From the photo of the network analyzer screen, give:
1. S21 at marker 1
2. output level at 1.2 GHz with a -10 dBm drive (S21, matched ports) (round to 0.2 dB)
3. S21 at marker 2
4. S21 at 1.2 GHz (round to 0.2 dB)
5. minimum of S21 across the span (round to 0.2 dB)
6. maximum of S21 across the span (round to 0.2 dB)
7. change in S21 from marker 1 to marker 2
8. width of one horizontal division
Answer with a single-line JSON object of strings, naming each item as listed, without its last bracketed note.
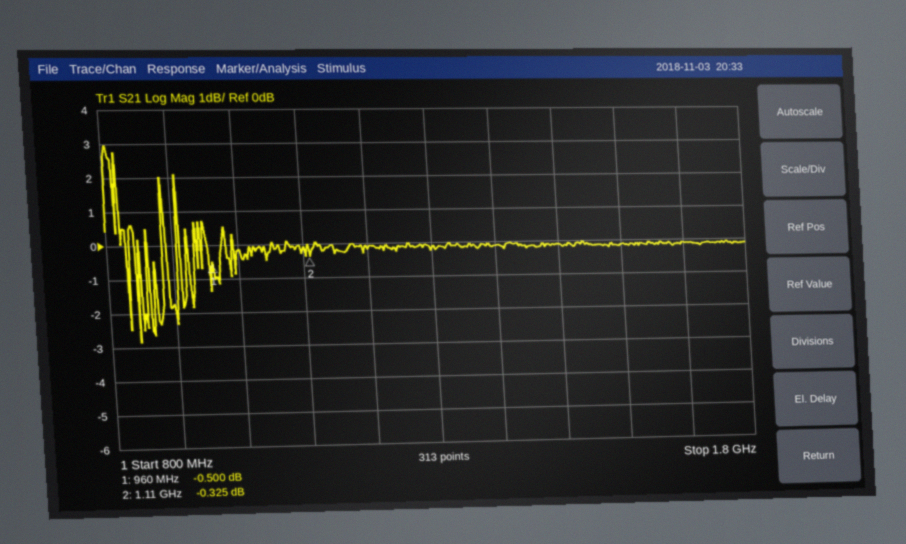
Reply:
{"S21 at marker 1": "-0.500 dB", "output level at 1.2 GHz with a -10 dBm drive (S21, matched ports)": "-10.2 dBm", "S21 at marker 2": "-0.325 dB", "S21 at 1.2 GHz": "-0.2 dB", "minimum of S21 across the span": "-2.8 dB", "maximum of S21 across the span": "3.0 dB", "change in S21 from marker 1 to marker 2": "0.175 dB", "width of one horizontal division": "100 MHz"}
